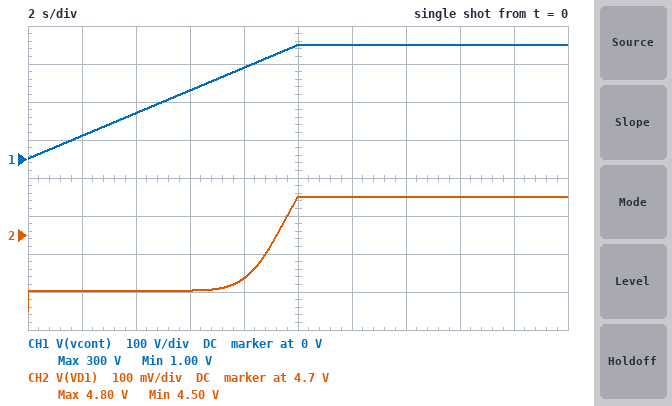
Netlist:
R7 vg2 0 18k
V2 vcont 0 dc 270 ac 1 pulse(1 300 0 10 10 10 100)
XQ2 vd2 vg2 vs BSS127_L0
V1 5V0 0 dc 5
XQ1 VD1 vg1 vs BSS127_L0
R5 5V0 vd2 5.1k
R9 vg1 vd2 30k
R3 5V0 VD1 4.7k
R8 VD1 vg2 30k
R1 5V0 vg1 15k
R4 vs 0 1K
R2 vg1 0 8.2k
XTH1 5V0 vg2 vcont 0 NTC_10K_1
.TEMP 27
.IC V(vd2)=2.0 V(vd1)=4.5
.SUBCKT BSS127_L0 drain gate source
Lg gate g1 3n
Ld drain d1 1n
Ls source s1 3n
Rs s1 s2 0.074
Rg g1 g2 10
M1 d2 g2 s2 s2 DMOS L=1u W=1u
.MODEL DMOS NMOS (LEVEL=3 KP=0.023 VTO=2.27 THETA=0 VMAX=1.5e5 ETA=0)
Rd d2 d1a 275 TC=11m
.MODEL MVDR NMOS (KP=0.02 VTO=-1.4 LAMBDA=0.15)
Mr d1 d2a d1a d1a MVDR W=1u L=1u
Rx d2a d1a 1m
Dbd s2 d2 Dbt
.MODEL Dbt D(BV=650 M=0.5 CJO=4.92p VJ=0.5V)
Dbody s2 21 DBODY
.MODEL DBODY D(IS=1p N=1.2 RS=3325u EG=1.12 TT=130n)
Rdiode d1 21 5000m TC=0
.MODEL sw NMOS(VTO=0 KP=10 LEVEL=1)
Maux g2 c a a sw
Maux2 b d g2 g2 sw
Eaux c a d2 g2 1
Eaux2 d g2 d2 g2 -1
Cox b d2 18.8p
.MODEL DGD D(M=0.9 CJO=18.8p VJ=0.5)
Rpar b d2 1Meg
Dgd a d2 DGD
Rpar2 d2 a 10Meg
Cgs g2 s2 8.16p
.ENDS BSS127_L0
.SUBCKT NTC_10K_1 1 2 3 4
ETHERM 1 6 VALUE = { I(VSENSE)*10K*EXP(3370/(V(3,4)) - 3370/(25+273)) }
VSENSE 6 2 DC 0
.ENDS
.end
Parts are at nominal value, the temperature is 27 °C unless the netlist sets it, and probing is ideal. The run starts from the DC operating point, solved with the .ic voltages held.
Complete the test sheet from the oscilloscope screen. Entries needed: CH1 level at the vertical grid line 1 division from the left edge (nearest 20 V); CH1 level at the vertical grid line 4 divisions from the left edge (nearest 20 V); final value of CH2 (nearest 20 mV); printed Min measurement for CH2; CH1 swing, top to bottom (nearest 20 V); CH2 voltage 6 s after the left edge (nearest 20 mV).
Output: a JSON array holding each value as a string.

["60 V", "240 V", "4.80 V", "4.50 V", "300 V", "4.56 V"]
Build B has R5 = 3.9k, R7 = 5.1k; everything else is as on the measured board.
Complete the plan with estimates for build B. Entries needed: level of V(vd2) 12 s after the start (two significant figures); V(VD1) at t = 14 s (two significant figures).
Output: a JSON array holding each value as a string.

["4.7 V", "4.6 V"]
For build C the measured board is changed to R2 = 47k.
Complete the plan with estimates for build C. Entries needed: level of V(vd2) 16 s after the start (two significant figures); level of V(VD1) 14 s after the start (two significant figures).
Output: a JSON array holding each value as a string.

["4.9 V", "1.2 V"]
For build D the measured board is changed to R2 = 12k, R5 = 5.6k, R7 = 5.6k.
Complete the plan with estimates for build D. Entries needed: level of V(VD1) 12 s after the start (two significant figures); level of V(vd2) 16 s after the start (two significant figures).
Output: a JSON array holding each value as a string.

["3.6 V", "4.6 V"]
